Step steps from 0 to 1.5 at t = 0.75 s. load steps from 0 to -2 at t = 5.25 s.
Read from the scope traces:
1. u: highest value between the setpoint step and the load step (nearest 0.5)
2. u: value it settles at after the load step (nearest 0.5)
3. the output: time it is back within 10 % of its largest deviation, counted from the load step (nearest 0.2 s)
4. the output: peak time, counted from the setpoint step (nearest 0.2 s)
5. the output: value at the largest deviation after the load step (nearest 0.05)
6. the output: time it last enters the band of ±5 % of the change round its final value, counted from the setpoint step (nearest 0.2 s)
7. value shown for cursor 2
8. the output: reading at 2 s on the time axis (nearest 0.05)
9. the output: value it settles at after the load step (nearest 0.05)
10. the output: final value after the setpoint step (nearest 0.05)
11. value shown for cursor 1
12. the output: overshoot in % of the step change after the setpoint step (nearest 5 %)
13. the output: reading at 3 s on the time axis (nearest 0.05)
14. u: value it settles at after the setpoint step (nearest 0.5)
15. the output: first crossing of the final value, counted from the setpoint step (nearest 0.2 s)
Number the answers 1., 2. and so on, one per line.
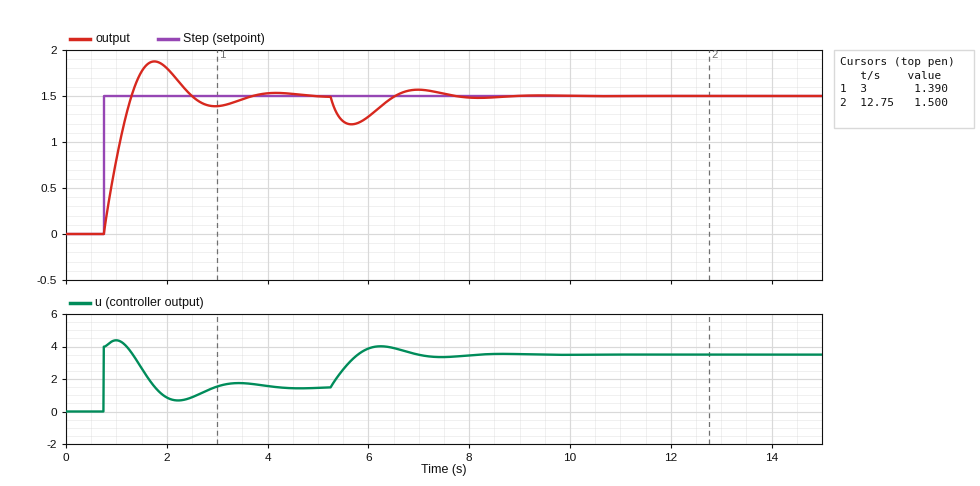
1. 4.5
2. 3.5
3. 2.2 s
4. 1.0 s
5. 1.20
6. 2.6 s
7. 1.500
8. 1.80
9. 1.50
10. 1.50
11. 1.390
12. 25 %
13. 1.40
14. 1.5
15. 0.6 s
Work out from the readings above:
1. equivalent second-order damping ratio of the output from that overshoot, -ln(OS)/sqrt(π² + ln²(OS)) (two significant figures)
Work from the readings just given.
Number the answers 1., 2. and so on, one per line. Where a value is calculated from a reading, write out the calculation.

1. ln(0.25) = -1.386; 1.386 / sqrt(9.870 + 1.922) = 0.40
